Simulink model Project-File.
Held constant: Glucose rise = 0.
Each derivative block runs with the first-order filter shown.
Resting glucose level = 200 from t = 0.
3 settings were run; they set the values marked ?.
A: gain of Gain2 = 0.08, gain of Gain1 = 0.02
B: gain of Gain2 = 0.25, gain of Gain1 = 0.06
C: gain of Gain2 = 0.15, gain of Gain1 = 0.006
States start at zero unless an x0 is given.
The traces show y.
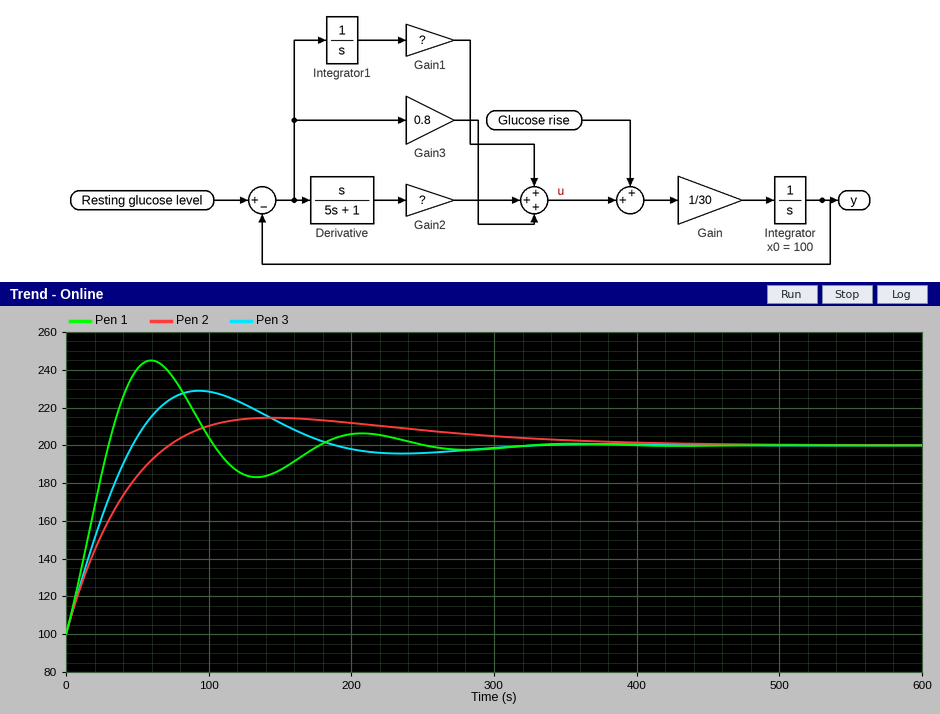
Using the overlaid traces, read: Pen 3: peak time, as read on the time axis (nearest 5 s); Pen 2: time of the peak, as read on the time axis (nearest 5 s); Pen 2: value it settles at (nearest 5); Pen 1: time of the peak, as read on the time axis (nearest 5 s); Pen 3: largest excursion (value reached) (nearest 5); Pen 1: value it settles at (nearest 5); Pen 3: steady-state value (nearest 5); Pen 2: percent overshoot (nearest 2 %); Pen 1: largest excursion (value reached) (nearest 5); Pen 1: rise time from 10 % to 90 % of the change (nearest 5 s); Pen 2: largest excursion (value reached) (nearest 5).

95 s
145 s
200
60 s
230
200
200
14 %
245
25 s
215
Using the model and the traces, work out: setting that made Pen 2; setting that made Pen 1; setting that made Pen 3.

C
B
A
